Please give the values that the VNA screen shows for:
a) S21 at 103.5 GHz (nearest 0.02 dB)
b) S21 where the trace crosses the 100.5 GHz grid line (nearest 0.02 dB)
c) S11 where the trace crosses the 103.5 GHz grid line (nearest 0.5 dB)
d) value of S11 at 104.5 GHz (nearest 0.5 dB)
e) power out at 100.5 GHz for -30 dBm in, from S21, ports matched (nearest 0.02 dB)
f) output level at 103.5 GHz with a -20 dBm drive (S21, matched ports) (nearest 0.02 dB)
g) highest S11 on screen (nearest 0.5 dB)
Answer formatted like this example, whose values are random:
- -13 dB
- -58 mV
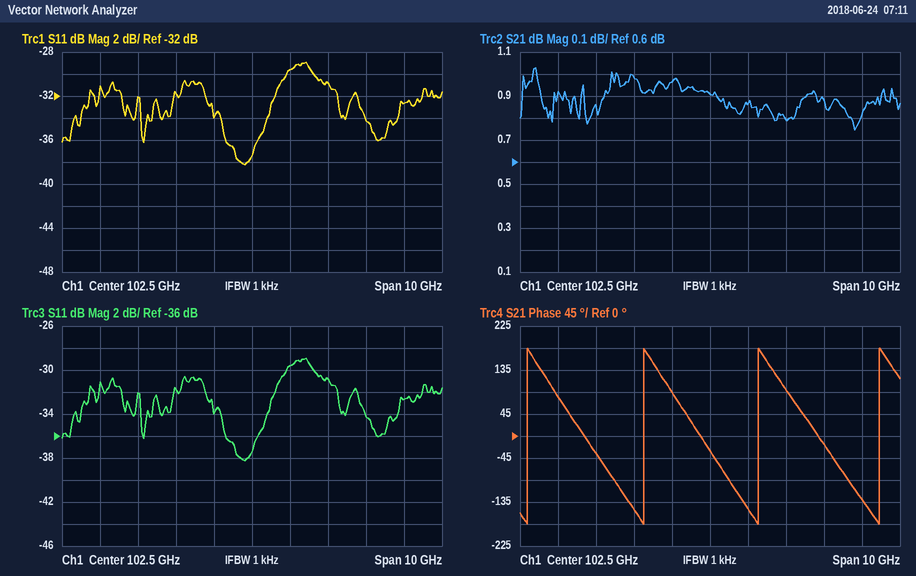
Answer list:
- 0.86 dB
- 0.98 dB
- -29.5 dB
- -31.0 dB
- -29.02 dBm
- -19.14 dBm
- -29.0 dB
